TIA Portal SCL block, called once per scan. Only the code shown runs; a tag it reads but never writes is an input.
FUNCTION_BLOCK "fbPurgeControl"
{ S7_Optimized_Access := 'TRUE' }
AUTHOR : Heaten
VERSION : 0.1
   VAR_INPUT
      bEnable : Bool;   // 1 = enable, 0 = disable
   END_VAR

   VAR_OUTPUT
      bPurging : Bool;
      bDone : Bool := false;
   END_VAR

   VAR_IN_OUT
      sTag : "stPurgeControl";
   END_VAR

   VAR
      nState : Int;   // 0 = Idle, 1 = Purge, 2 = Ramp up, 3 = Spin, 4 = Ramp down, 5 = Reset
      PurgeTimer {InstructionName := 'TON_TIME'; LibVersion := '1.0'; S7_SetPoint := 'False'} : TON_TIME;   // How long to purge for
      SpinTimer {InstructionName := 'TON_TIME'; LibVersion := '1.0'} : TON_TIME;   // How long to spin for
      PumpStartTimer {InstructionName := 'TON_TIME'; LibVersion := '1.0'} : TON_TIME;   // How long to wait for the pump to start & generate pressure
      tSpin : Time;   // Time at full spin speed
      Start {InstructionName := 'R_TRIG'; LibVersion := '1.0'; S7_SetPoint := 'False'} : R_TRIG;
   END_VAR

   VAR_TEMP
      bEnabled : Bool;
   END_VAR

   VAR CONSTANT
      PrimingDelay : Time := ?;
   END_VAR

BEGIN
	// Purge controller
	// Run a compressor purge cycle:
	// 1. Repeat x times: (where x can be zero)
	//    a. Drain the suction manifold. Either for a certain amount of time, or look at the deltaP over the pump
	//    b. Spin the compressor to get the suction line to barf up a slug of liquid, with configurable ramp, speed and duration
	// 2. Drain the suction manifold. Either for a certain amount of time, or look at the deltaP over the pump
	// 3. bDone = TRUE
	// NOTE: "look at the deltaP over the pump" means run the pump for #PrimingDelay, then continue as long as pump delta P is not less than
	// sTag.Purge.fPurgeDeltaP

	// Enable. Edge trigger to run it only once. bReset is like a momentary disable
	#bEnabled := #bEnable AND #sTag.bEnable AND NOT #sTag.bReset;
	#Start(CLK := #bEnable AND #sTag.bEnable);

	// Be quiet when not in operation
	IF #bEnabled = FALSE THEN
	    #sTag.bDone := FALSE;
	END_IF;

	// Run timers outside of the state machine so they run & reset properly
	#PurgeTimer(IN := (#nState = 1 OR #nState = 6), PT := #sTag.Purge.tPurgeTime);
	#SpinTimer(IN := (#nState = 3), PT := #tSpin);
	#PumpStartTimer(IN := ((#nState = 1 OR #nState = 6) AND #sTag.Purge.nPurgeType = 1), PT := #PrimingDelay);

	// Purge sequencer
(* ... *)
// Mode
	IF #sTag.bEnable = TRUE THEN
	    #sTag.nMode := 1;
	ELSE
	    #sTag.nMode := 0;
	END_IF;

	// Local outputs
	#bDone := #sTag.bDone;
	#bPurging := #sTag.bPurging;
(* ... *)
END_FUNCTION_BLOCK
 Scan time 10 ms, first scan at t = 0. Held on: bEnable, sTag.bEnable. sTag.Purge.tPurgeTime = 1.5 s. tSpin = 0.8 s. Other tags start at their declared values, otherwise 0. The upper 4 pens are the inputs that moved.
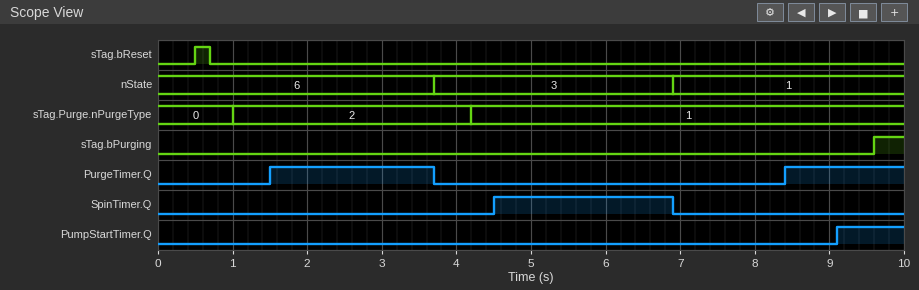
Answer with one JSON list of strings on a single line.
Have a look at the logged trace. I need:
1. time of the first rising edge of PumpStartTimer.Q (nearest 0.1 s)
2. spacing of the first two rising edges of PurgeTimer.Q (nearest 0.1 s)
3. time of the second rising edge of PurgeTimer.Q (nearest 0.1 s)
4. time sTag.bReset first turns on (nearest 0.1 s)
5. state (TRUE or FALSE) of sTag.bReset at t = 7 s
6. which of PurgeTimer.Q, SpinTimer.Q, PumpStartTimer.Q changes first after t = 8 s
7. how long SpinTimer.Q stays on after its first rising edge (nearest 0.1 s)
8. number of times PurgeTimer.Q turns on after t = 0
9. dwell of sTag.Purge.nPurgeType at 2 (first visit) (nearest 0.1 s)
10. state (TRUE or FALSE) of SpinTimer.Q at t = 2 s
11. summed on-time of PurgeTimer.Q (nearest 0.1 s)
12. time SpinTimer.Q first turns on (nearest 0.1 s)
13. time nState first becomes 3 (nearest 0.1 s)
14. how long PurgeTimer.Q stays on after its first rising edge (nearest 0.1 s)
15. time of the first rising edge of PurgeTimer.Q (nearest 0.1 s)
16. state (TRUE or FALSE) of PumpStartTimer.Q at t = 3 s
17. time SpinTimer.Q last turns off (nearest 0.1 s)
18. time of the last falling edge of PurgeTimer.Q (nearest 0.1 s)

["9.1 s", "6.9 s", "8.4 s", "0.5 s", "FALSE", "PurgeTimer.Q", "2.4 s", "2", "3.2 s", "FALSE", "3.8 s", "4.5 s", "3.7 s", "2.2 s", "1.5 s", "FALSE", "6.9 s", "3.7 s"]
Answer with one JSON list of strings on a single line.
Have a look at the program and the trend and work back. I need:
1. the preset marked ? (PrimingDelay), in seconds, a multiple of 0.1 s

["2.2 s"]
